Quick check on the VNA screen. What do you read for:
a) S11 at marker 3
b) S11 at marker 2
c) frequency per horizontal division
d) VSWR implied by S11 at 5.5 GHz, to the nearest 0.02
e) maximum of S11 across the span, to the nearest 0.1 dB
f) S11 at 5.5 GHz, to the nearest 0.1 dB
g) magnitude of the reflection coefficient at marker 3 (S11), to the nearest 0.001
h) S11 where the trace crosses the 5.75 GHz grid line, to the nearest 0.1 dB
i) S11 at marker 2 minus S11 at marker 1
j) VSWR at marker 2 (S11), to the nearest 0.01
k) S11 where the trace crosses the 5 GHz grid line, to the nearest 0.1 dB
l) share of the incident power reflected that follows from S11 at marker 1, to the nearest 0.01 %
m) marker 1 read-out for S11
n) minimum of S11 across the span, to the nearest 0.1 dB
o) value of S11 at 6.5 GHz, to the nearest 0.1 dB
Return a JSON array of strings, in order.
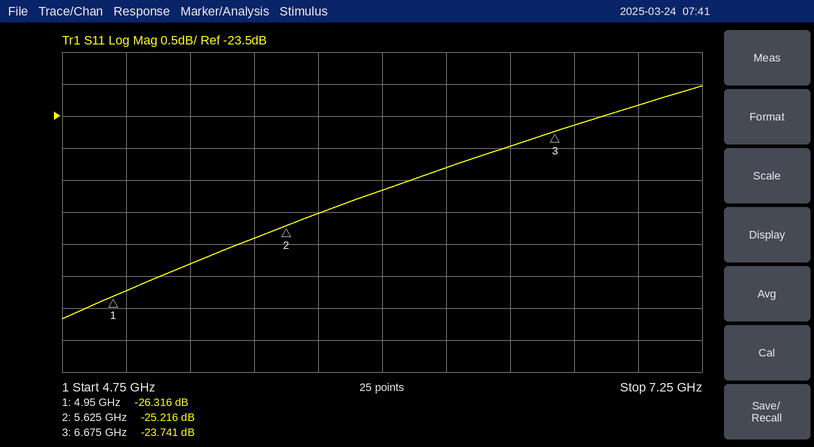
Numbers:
["-23.741 dB", "-25.216 dB", "250 MHz", "1.12", "-23.0 dB", "-25.4 dB", "0.065", "-25.0 dB", "1.100 dB", "1.12", "-26.2 dB", "0.23 %", "-26.316 dB", "-26.7 dB", "-24.0 dB"]
